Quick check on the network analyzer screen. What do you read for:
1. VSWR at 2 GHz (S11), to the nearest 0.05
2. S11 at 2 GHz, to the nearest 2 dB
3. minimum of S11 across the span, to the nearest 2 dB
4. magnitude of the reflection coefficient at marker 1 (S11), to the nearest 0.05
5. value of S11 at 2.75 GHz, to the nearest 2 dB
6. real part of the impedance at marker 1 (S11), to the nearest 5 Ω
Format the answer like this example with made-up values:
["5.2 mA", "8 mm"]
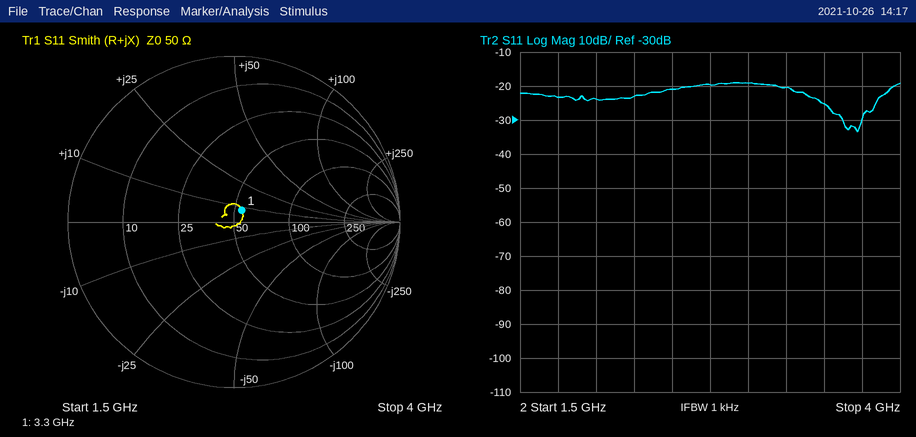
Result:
["1.15", "-24 dB", "-34 dB", "0.10", "-20 dB", "55 Ω"]
